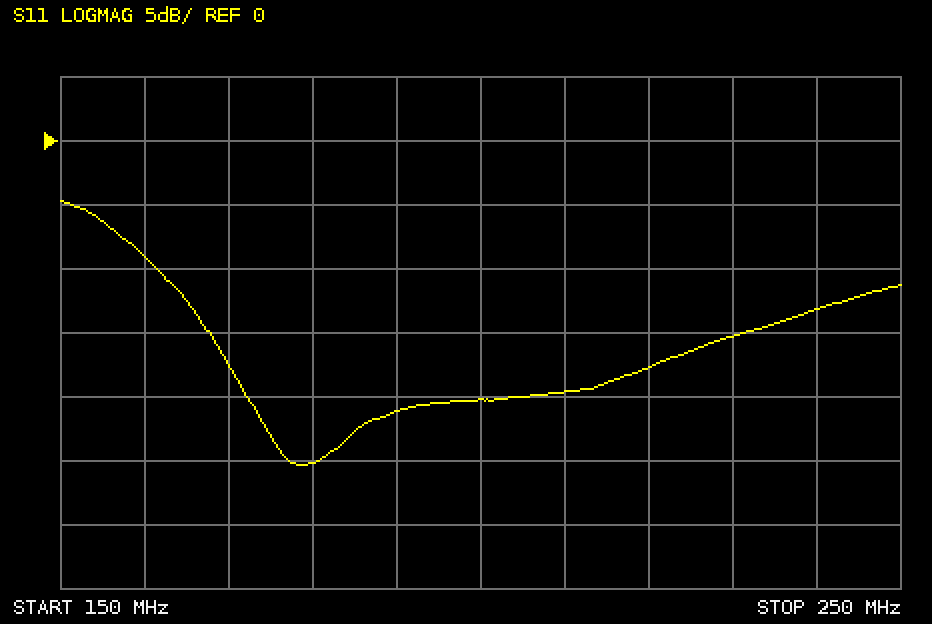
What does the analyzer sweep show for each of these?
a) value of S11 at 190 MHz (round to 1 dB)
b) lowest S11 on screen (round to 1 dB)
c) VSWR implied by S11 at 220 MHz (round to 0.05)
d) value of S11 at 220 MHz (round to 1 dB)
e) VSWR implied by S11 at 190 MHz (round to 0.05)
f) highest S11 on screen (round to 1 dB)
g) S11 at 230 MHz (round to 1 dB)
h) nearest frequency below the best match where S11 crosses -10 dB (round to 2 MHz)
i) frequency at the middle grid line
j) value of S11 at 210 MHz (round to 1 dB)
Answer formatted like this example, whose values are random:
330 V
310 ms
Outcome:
-21 dB
-25 dB
1.30
-18 dB
1.20
-5 dB
-15 dB
162 MHz
200 MHz
-20 dB
